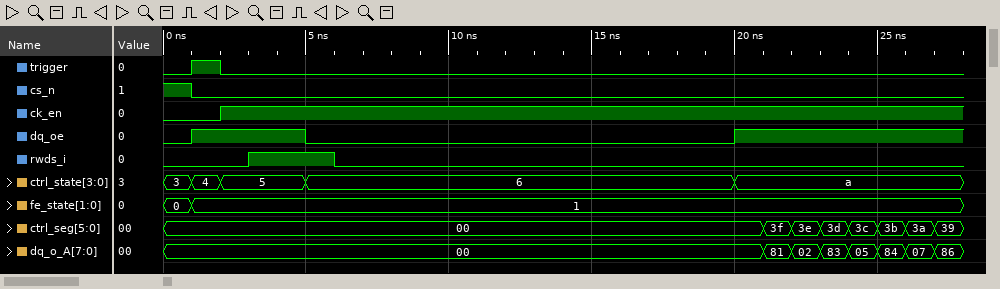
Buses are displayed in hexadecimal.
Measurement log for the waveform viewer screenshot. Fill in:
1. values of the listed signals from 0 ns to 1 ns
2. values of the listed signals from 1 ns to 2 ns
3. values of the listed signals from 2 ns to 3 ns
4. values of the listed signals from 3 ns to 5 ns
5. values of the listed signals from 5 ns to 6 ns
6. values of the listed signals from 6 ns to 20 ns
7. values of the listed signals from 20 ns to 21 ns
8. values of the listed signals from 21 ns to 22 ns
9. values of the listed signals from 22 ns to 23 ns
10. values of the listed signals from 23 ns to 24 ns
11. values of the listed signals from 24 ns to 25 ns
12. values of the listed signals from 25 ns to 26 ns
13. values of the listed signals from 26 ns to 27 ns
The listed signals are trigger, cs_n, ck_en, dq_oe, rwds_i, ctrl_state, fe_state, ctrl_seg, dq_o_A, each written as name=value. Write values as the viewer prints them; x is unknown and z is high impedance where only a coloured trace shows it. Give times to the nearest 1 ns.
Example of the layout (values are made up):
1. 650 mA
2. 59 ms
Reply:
1. trigger=0, cs_n=1, ck_en=0, dq_oe=0, rwds_i=0, ctrl_state=3, fe_state=0, ctrl_seg=00, dq_o_A=00
2. trigger=1, cs_n=0, ck_en=0, dq_oe=1, rwds_i=0, ctrl_state=4, fe_state=1, ctrl_seg=00, dq_o_A=00
3. trigger=0, cs_n=0, ck_en=1, dq_oe=1, rwds_i=0, ctrl_state=5, fe_state=1, ctrl_seg=00, dq_o_A=00
4. trigger=0, cs_n=0, ck_en=1, dq_oe=1, rwds_i=1, ctrl_state=5, fe_state=1, ctrl_seg=00, dq_o_A=00
5. trigger=0, cs_n=0, ck_en=1, dq_oe=0, rwds_i=1, ctrl_state=6, fe_state=1, ctrl_seg=00, dq_o_A=00
6. trigger=0, cs_n=0, ck_en=1, dq_oe=0, rwds_i=0, ctrl_state=6, fe_state=1, ctrl_seg=00, dq_o_A=00
7. trigger=0, cs_n=0, ck_en=1, dq_oe=1, rwds_i=0, ctrl_state=a, fe_state=1, ctrl_seg=00, dq_o_A=00
8. trigger=0, cs_n=0, ck_en=1, dq_oe=1, rwds_i=0, ctrl_state=a, fe_state=1, ctrl_seg=3f, dq_o_A=81
9. trigger=0, cs_n=0, ck_en=1, dq_oe=1, rwds_i=0, ctrl_state=a, fe_state=1, ctrl_seg=3e, dq_o_A=02
10. trigger=0, cs_n=0, ck_en=1, dq_oe=1, rwds_i=0, ctrl_state=a, fe_state=1, ctrl_seg=3d, dq_o_A=83
11. trigger=0, cs_n=0, ck_en=1, dq_oe=1, rwds_i=0, ctrl_state=a, fe_state=1, ctrl_seg=3c, dq_o_A=05
12. trigger=0, cs_n=0, ck_en=1, dq_oe=1, rwds_i=0, ctrl_state=a, fe_state=1, ctrl_seg=3b, dq_o_A=84
13. trigger=0, cs_n=0, ck_en=1, dq_oe=1, rwds_i=0, ctrl_state=a, fe_state=1, ctrl_seg=3a, dq_o_A=07
